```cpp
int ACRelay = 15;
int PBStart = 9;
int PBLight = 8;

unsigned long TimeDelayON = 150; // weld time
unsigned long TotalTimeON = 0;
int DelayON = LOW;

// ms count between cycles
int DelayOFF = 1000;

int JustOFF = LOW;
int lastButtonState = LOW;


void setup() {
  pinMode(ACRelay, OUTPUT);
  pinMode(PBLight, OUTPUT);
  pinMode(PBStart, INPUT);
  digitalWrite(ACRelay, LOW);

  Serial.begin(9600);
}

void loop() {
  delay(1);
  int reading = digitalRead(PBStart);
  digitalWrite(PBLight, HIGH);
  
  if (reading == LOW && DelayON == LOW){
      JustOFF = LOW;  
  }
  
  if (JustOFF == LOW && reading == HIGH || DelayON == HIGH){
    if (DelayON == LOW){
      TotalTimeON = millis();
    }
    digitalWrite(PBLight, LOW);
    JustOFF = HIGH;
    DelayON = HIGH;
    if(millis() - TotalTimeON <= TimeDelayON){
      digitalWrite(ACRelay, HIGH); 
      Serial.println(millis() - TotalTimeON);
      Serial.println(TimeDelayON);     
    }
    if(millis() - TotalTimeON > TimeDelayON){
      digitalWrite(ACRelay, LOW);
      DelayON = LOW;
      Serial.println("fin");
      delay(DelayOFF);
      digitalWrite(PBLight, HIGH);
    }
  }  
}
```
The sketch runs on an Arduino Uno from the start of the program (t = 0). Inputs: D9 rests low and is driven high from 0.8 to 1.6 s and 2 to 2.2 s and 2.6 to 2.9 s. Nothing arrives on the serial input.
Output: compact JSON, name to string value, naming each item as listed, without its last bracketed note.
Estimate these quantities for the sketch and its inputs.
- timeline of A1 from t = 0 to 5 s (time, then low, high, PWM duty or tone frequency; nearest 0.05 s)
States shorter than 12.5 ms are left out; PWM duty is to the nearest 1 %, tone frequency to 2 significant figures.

{"timeline of A1 from t = 0 to 5 s": "0 s low; 0.8 s high; 0.95 s low; 2 s high; 2.15 s low"}
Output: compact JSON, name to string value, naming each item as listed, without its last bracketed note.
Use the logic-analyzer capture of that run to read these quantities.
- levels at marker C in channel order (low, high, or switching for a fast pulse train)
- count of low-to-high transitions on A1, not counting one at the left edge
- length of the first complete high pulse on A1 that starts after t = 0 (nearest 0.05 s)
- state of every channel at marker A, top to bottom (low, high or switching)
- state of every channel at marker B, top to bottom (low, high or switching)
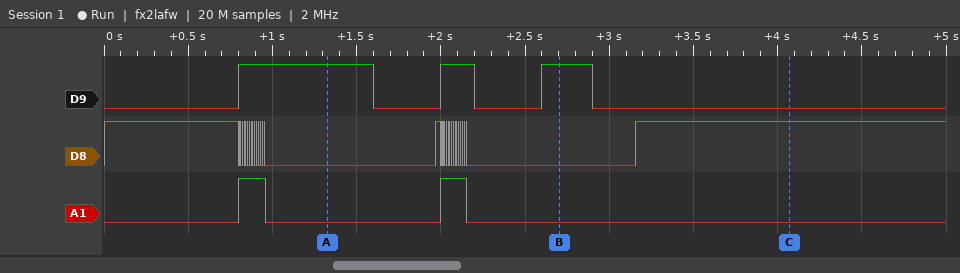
{"levels at marker C in channel order": "D9 low, D8 high, A1 low", "count of low-to-high transitions on A1, not counting one at the left edge": "2", "length of the first complete high pulse on A1 that starts after t = 0": "0.15 s", "state of every channel at marker A, top to bottom": "D9 high, D8 low, A1 low", "state of every channel at marker B, top to bottom": "D9 high, D8 low, A1 low"}
